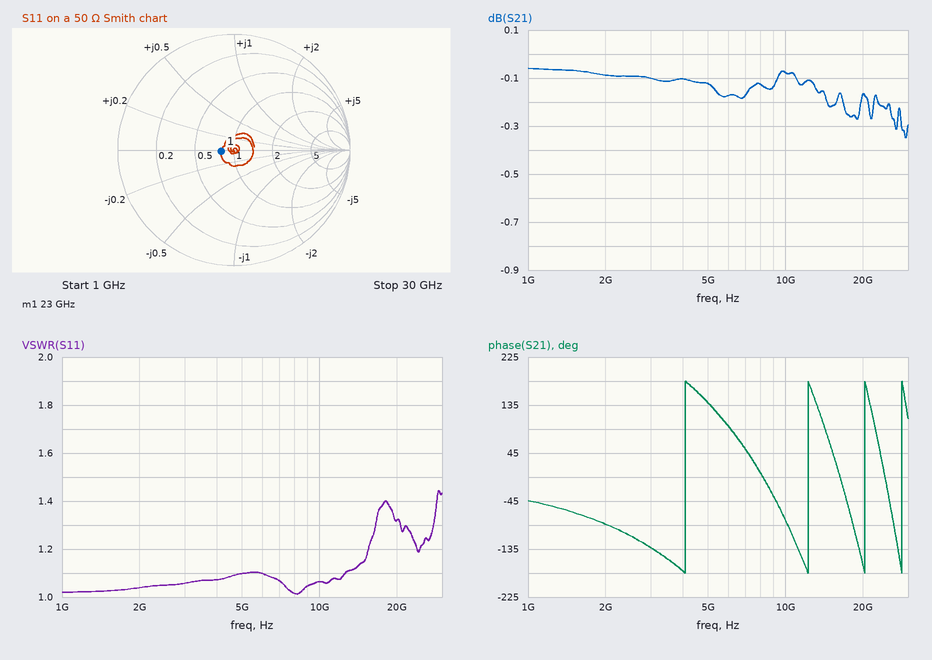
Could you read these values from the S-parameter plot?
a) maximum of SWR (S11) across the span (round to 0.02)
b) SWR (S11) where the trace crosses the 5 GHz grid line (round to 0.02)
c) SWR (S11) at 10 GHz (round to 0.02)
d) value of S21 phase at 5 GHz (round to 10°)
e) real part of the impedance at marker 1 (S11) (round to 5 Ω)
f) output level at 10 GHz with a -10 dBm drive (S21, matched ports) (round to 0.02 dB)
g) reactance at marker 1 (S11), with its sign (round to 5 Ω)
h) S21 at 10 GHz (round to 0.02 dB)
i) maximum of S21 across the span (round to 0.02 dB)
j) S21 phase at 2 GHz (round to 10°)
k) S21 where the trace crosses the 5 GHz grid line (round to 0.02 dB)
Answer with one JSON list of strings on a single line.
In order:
["1.44", "1.10", "1.06", "140°", "40 Ω", "-10.08 dBm", "0 Ω", "-0.08 dB", "-0.06 dB", "-90°", "-0.12 dB"]
